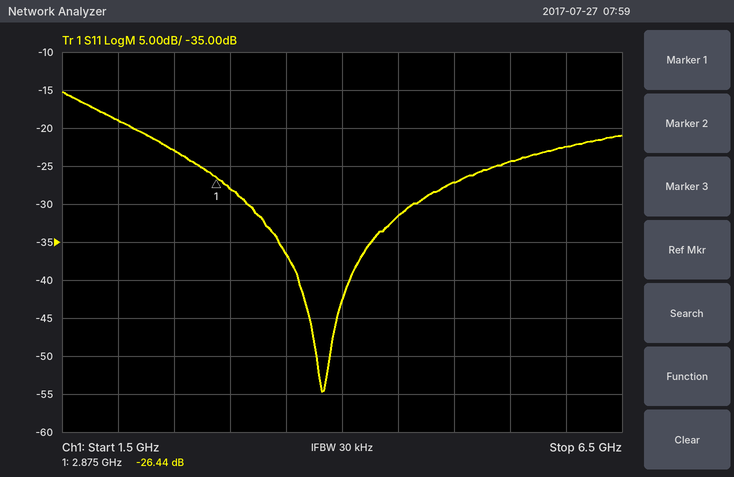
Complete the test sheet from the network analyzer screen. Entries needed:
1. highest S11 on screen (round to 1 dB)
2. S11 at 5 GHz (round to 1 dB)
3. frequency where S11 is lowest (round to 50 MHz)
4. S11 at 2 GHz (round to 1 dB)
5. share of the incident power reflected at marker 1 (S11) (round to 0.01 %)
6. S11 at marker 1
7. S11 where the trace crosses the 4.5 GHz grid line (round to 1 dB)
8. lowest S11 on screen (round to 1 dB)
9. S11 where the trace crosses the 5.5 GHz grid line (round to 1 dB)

-15 dB
-27 dB
3.80 GHz
-19 dB
0.23 %
-26.44 dB
-32 dB
-55 dB
-24 dB
